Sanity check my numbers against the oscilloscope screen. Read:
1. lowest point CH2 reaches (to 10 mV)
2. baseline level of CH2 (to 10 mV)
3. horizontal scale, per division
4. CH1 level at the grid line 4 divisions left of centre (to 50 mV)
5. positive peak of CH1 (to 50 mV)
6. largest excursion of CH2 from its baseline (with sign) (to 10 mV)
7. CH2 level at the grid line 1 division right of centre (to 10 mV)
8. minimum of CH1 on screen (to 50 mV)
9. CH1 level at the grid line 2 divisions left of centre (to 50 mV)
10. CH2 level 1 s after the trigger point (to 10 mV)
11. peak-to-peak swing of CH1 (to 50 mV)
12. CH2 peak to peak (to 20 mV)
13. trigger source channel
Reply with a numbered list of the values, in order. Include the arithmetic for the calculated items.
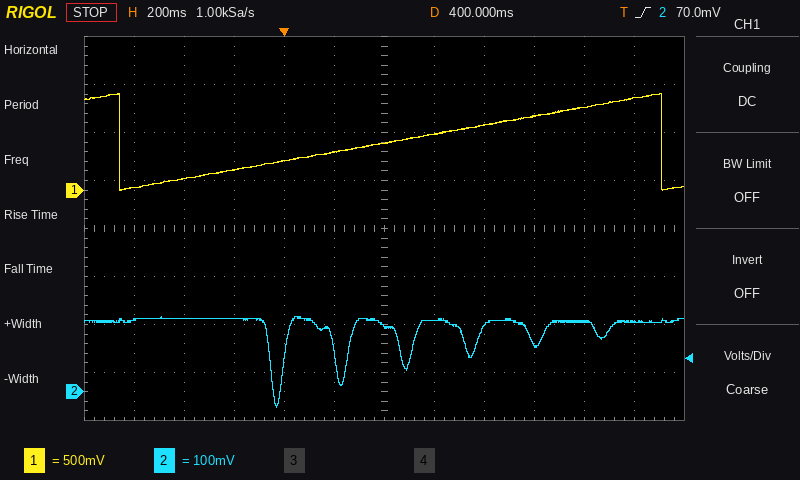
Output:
1. -30 mV
2. 150 mV
3. 200 ms
4. 100 mV
5. 1.00 V
6. -30 mV − (150 mV) = -180 mV
7. 150 mV
8. 0 mV
9. 300 mV
10. 100 mV
11. 1.00 V − (0 mV) = 1.00 V
12. 180 mV
13. CH2
